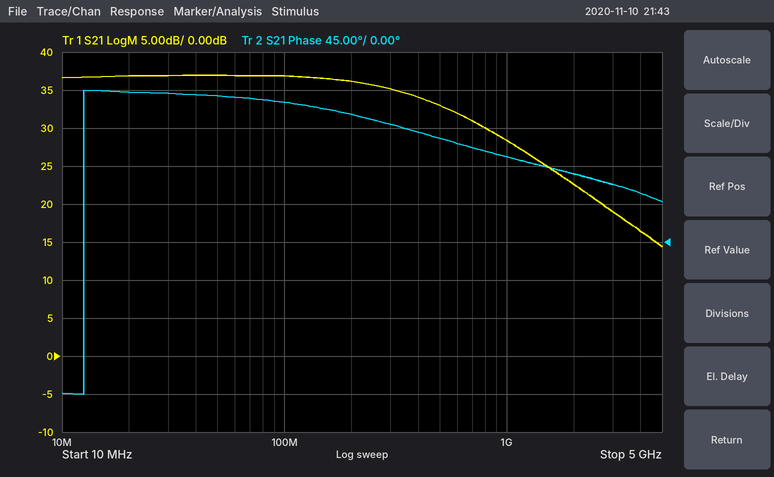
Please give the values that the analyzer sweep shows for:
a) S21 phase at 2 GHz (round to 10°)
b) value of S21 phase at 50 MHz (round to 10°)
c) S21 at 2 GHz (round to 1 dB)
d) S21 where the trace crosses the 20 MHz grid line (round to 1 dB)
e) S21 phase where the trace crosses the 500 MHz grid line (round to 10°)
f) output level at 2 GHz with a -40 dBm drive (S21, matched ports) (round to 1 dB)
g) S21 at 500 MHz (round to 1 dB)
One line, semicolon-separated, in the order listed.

80°; 170°; 23 dB; 37 dB; 120°; -17 dBm; 33 dB
